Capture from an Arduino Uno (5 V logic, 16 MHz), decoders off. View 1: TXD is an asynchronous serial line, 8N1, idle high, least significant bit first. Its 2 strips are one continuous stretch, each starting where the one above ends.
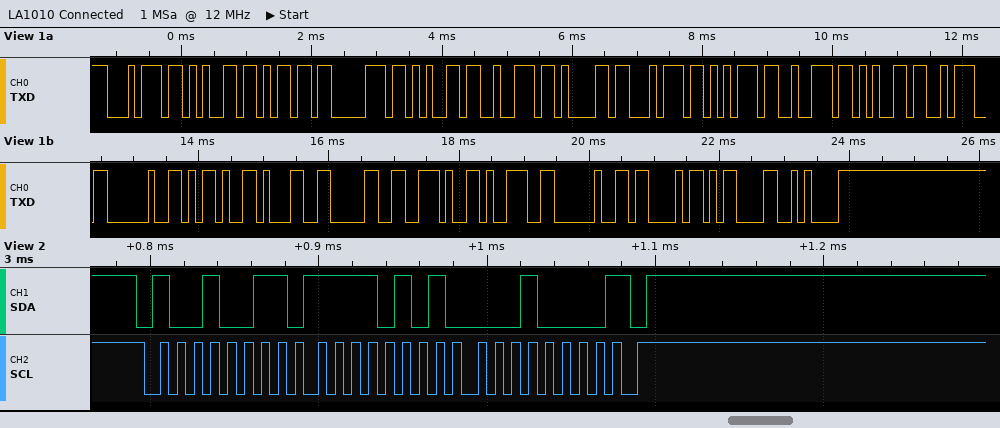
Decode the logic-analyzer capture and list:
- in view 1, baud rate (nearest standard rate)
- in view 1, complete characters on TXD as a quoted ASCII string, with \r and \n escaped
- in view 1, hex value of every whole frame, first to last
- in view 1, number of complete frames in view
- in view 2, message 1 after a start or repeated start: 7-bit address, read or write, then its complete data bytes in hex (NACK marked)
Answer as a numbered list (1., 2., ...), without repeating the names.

1. 9600 baud
2. "temperature: -10.9 C\r\n"
3. 74 65 6D 70 65 72 61 74 75 72 65 3A 20 2D 31 30 2E 39 20 43 0D 0A
4. 22
5. 0x49 read: F5 10 NACK
